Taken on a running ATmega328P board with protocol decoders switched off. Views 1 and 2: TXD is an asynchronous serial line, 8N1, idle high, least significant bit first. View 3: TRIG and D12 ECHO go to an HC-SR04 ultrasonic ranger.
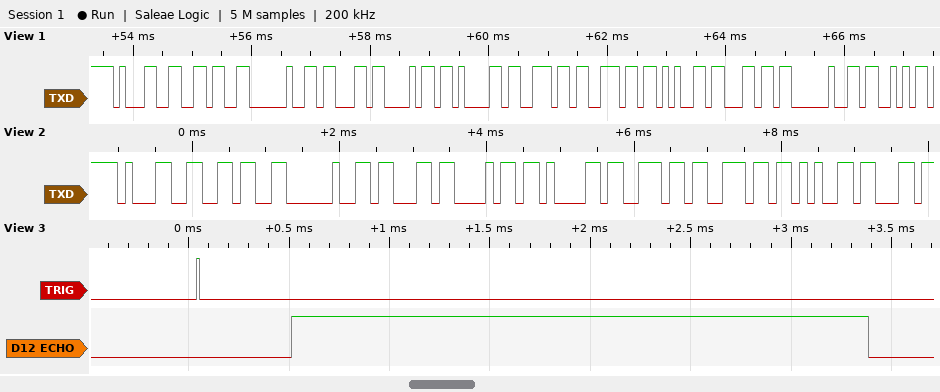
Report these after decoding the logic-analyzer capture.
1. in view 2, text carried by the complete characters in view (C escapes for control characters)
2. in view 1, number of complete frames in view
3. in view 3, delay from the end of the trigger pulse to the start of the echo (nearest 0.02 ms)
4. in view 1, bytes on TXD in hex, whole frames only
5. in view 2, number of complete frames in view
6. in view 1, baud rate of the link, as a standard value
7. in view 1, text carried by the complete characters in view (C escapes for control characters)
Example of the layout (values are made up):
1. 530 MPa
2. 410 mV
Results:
1. "16 channe"
2. 12
3. 0.46 ms
4. 0x31 0x36 0x20 0x63 0x68 0x61 0x6E 0x6E 0x65 0x6C 0x20 0x53
5. 9
6. 9600 baud
7. "16 channel S"
